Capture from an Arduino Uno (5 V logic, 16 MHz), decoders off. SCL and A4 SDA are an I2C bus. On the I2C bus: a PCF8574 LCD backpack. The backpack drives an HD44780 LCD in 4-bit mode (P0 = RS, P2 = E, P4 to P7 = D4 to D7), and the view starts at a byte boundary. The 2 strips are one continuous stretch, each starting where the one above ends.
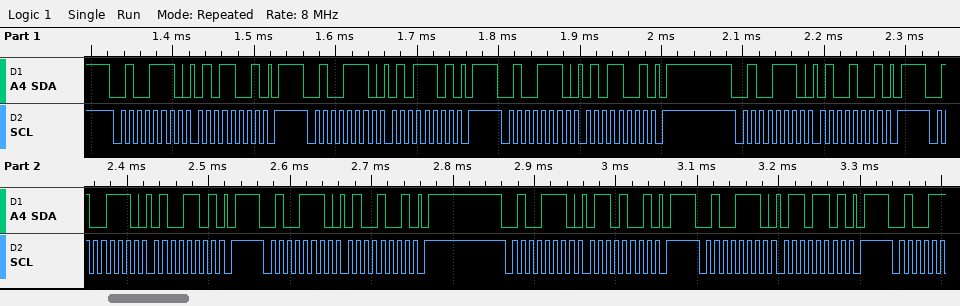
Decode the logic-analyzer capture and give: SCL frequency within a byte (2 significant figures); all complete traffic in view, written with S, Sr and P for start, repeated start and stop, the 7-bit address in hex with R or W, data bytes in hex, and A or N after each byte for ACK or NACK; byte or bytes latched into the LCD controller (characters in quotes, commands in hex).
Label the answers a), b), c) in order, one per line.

a) 100 kHz
b) S 27W A 59 A P S 27W A 5D A P S 27W A 59 A P S 27W A 49 A P S 27W A 4D A P S 27W A 49 A P S 27W A 69 A P S 27W A 6D A P
c) 'T'
